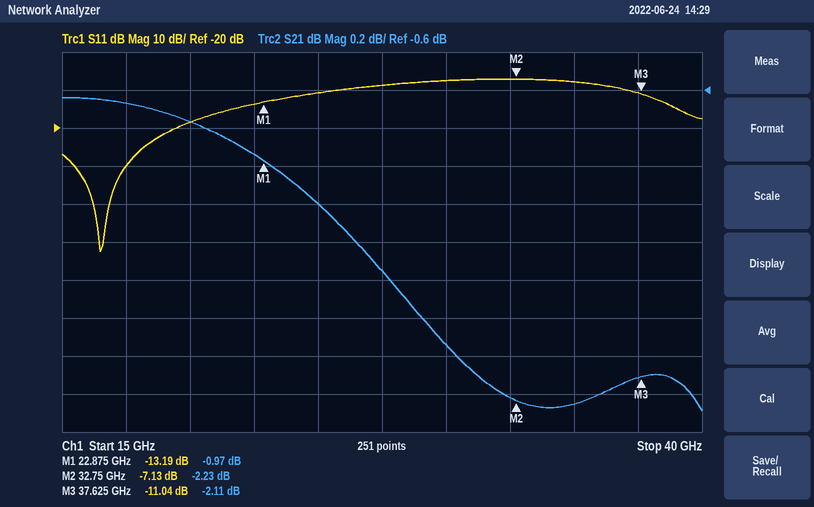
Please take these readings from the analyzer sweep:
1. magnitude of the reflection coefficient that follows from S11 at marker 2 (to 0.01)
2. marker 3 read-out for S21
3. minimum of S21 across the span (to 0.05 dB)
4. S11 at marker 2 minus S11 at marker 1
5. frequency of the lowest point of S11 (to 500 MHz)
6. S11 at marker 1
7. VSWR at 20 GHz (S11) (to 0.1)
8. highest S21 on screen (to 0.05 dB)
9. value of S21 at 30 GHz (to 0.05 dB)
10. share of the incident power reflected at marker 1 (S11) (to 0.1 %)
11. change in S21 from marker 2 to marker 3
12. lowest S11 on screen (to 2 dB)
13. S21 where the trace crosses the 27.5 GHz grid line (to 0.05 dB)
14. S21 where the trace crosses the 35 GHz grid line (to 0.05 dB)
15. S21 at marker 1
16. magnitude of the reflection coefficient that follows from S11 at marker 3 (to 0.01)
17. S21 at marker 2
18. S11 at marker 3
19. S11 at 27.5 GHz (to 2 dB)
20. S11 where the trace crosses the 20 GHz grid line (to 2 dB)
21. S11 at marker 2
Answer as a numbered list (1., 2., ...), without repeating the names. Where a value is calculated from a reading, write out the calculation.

1. 10^(-7.13/20) ≈ 0.44
2. -2.11 dB
3. -2.30 dB
4. -7.13 − (-13.19) = 6.06 dB
5. 16.5 GHz
6. -13.19 dB
7. |Γ| = 10^(-18/20) = 0.1259; VSWR = (1 + 0.1259)/(1 − 0.1259) ≈ 1.3
8. -0.65 dB
9. -1.95 dB
10. 10^(-13.19/10) ≈ 4.8 %
11. -2.11 − (-2.23) = 0.12 dB
12. -52 dB
13. -1.55 dB
14. -2.25 dB
15. -0.97 dB
16. 10^(-11.04/20) ≈ 0.28
17. -2.23 dB
18. -11.04 dB
19. -8 dB
20. -18 dB
21. -7.13 dB
